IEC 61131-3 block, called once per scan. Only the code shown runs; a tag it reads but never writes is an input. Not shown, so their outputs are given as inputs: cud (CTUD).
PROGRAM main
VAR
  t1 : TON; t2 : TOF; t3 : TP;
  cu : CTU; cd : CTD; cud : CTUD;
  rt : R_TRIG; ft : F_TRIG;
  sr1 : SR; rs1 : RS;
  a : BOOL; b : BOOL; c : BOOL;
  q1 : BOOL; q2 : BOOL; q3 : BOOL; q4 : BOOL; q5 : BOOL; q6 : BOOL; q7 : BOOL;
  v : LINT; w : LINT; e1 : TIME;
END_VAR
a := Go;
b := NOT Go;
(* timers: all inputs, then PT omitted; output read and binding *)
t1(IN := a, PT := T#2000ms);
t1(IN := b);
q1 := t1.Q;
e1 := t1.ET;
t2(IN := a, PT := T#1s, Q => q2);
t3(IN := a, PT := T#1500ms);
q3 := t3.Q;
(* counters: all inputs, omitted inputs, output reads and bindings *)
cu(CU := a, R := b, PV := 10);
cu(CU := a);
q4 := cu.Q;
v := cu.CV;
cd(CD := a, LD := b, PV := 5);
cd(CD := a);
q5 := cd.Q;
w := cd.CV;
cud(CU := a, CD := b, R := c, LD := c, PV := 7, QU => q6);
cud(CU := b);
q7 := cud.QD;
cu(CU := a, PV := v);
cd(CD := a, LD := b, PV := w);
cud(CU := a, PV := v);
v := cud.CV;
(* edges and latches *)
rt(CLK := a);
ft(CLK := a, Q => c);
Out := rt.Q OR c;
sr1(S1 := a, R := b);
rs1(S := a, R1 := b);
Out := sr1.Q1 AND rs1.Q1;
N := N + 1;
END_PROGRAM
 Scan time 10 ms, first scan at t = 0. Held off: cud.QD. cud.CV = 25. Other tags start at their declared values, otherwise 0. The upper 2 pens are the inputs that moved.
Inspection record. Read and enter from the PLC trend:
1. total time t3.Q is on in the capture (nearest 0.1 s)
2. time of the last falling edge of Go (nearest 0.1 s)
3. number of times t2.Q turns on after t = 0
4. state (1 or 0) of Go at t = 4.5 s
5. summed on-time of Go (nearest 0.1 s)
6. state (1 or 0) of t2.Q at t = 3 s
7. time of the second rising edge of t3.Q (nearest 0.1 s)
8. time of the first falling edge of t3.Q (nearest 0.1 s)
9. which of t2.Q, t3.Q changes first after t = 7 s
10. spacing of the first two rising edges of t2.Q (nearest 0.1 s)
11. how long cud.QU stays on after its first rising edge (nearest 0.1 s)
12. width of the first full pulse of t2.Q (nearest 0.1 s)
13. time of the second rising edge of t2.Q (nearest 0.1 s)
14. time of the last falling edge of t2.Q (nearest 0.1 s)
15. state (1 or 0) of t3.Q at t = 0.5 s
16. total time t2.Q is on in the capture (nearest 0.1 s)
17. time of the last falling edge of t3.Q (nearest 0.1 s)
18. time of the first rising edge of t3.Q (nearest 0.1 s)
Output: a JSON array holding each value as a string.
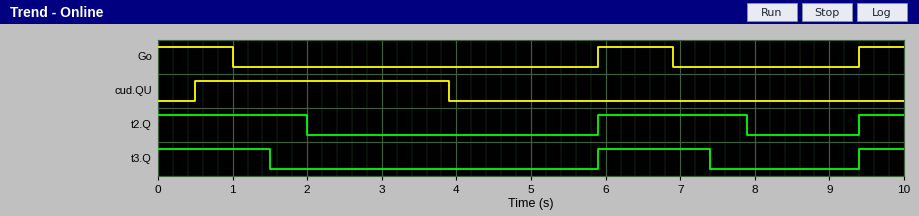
["3.6 s", "6.9 s", "2", "0", "2.6 s", "0", "9.4 s", "1.5 s", "t3.Q", "3.5 s", "3.4 s", "2.0 s", "9.4 s", "7.9 s", "1", "4.6 s", "7.4 s", "5.9 s"]
